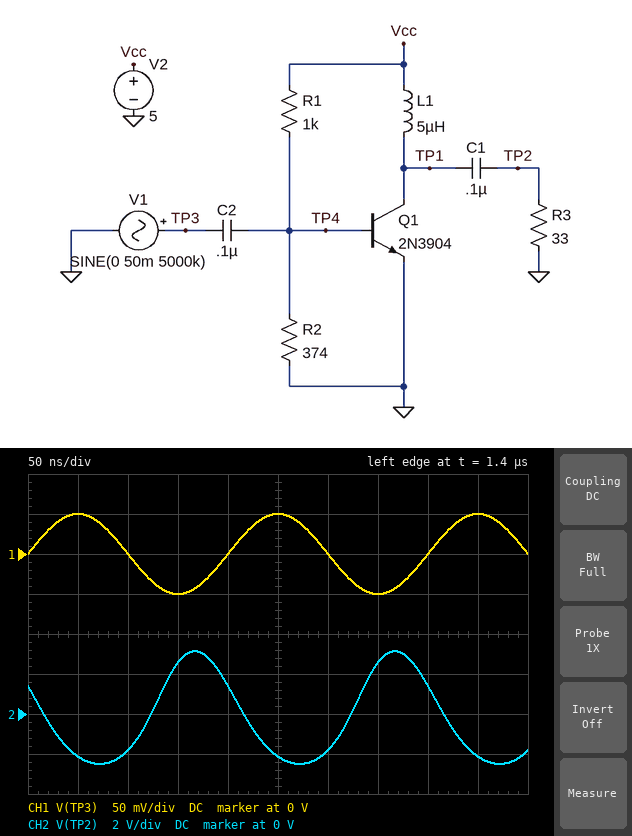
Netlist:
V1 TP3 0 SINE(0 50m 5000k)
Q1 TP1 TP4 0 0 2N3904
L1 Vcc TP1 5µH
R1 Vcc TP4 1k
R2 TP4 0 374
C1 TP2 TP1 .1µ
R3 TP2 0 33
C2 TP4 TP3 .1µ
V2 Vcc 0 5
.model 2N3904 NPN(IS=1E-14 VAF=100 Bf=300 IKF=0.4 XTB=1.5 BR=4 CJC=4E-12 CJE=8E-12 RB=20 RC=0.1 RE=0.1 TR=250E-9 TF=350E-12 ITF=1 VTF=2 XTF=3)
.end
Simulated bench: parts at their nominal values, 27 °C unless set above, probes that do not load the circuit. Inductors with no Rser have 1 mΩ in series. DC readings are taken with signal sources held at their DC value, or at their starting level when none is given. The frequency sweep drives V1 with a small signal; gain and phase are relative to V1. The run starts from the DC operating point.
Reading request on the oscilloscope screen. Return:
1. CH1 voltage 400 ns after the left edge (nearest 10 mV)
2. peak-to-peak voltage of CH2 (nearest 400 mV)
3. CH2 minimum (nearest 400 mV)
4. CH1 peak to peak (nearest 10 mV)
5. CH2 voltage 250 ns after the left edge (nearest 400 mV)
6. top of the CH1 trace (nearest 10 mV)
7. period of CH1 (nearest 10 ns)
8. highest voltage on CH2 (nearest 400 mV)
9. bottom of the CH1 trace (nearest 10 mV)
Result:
0 V
5.6 V
-2.4 V
100 mV
-2.0 V
50 mV
200 ns
3.2 V
-50 mV
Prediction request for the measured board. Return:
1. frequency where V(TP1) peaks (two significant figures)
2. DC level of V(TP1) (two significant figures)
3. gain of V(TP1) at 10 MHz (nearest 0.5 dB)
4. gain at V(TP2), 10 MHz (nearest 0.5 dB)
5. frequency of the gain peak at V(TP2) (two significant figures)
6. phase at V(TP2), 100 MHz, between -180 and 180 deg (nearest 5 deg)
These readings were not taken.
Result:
2.2 MHz
5.0 V
31.5 dB
31.5 dB
2.2 MHz
90 deg
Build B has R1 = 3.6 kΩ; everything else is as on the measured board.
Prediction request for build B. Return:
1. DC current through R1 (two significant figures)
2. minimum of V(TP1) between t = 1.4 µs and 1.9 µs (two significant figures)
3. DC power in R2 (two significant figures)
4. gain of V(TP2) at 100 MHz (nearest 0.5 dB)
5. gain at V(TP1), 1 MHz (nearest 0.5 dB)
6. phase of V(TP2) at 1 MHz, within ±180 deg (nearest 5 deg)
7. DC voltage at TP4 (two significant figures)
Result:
1.3 mA
5.0 V
590 µW
-27.5 dB
-62.0 dB
-155 deg
470 mV
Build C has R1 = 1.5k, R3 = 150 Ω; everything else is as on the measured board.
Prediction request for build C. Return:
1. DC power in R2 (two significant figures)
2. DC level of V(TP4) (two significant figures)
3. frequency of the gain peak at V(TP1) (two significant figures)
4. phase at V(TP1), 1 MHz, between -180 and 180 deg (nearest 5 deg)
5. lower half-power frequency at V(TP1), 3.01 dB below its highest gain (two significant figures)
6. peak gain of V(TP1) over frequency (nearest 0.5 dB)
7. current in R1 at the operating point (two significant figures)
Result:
1.8 mW
820 mV
4.7 MHz
-110 deg
2.2 MHz
46.0 dB
2.8 mA
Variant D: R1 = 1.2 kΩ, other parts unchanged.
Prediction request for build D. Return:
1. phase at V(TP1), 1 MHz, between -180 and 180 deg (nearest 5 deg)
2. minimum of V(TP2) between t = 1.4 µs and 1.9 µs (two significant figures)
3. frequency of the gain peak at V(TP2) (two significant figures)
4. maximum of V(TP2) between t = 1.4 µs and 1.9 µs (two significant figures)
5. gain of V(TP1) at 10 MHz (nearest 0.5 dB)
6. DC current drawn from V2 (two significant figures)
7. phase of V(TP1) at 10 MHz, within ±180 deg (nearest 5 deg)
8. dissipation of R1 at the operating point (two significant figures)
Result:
-145 deg
-2.7 V
2.4 MHz
3.2 V
32.5 dB
240 mA
125 deg
14 mW
